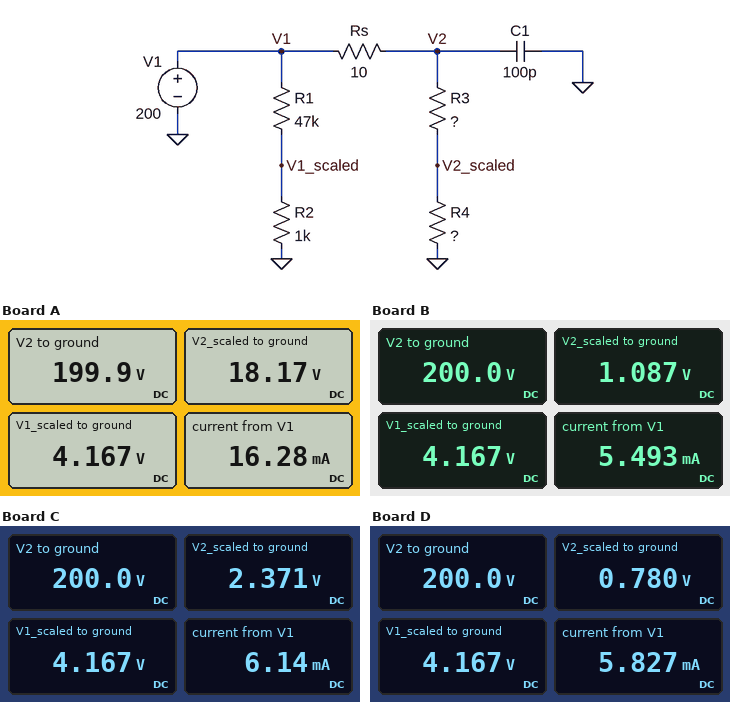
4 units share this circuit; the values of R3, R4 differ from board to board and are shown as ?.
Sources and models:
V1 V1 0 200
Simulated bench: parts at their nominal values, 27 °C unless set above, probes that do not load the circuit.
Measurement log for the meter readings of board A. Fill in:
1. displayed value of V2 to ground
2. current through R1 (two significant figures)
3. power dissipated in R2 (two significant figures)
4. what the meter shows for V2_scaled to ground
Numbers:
199.9 V
4.2 mA
17 mW
18.17 V
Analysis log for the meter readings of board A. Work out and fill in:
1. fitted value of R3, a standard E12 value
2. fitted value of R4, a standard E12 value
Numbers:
15 kΩ
1.5 kΩ
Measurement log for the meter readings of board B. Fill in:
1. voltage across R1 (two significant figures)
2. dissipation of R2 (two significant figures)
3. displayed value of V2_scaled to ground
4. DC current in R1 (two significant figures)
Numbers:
200 V
17 mW
1.087 V
4.2 mA
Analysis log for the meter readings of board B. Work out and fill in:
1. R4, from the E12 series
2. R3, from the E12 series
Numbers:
820 Ω
150 kΩ
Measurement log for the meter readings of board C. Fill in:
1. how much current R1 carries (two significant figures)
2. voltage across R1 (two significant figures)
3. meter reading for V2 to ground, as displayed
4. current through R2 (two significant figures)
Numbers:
4.2 mA
200 V
200.0 V
4.2 mA
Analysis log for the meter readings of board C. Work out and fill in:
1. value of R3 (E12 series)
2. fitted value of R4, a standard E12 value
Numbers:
100 kΩ
1.2 kΩ
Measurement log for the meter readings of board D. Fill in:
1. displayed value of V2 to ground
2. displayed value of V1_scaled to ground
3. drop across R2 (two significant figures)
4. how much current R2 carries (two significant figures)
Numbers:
200.0 V
4.167 V
4.2 V
4.2 mA
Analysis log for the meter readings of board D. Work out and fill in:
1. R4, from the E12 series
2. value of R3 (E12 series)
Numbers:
470 Ω
120 kΩ
